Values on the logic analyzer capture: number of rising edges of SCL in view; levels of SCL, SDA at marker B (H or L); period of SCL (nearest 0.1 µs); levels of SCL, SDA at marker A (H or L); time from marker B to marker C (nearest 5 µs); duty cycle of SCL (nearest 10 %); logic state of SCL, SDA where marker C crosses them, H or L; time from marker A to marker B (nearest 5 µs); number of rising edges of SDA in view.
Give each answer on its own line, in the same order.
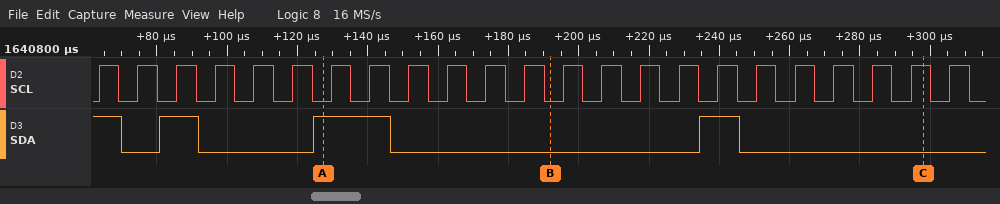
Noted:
23
SCL=L, SDA=L
11 µs
SCL=L, SDA=H
105 µs
50 %
SCL=H, SDA=L
65 µs
3
